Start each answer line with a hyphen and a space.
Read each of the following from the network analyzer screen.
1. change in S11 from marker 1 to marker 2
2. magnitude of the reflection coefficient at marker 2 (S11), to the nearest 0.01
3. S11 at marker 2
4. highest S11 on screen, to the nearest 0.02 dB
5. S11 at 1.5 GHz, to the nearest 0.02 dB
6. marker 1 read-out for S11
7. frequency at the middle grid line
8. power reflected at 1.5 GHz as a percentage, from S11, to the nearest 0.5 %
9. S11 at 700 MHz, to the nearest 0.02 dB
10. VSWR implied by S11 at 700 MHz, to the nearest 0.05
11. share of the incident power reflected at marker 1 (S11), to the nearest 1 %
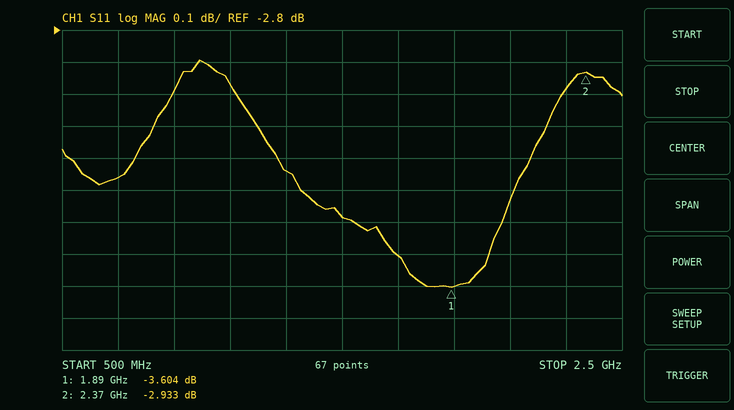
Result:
- 0.671 dB
- 0.71
- -2.933 dB
- -2.90 dB
- -3.38 dB
- -3.604 dB
- 1.5 GHz
- 46.0 %
- -3.26 dB
- 5.40
- 44 %
